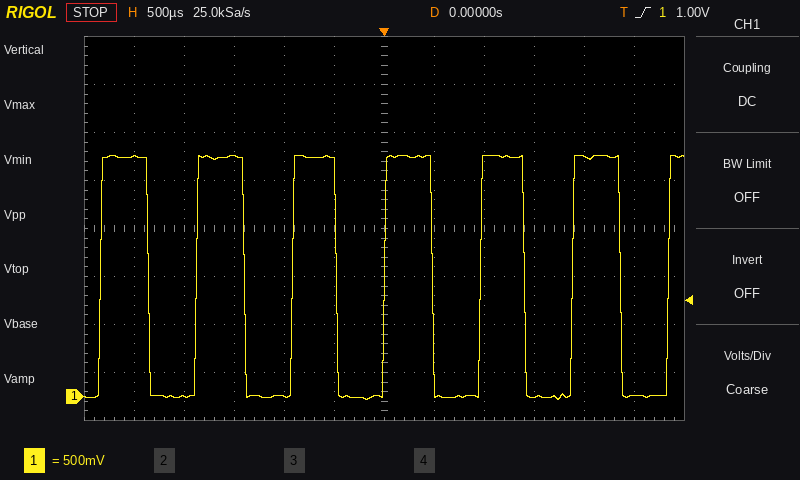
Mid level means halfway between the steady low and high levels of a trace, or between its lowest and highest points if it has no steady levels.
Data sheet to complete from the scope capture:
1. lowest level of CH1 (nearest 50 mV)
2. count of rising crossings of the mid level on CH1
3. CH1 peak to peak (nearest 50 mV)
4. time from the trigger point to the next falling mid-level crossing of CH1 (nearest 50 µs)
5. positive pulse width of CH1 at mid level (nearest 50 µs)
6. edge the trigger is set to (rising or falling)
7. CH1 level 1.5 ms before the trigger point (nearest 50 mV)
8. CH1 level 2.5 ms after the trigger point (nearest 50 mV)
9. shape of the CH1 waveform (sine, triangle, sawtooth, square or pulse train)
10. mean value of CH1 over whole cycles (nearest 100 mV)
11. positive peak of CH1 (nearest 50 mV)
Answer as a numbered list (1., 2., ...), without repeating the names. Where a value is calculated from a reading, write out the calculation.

1. -50 mV
2. 7
3. 2.50 V − (-50 mV) = 2.55 V
4. 500 µs
5. 450 µs
6. rising
7. 2.50 V
8. 0 mV
9. square
10. -50 mV + 0.5 × (2.50 V − (-50 mV)) ≈ 1.2 V
11. 2.50 V
